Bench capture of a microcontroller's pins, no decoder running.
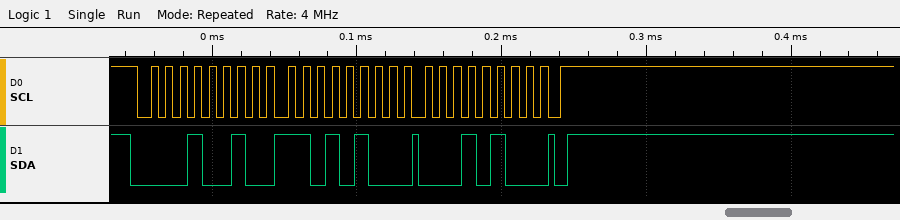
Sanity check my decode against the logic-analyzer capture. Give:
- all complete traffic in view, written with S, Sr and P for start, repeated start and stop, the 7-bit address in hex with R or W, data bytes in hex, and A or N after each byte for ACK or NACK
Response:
S 09W A D4 A 14 A P
